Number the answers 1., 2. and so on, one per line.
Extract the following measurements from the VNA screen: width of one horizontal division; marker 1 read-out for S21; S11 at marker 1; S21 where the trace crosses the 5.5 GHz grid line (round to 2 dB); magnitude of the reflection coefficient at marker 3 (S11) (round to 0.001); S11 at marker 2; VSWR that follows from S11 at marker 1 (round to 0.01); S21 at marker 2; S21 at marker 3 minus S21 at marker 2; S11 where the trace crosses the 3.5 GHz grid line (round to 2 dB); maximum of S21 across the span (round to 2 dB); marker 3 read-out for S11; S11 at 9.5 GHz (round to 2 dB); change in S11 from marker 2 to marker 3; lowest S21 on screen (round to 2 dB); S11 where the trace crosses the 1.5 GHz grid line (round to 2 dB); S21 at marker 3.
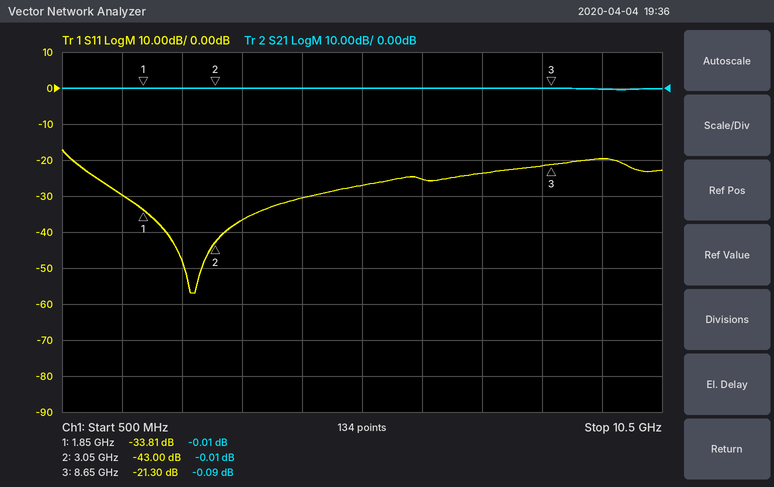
1. 1 GHz
2. -0.01 dB
3. -33.81 dB
4. 0 dB
5. 0.086
6. -43.00 dB
7. 1.04
8. -0.01 dB
9. -0.08 dB
10. -36 dB
11. 0 dB
12. -21.30 dB
13. -20 dB
14. 21.70 dB
15. 0 dB
16. -30 dB
17. -0.09 dB
